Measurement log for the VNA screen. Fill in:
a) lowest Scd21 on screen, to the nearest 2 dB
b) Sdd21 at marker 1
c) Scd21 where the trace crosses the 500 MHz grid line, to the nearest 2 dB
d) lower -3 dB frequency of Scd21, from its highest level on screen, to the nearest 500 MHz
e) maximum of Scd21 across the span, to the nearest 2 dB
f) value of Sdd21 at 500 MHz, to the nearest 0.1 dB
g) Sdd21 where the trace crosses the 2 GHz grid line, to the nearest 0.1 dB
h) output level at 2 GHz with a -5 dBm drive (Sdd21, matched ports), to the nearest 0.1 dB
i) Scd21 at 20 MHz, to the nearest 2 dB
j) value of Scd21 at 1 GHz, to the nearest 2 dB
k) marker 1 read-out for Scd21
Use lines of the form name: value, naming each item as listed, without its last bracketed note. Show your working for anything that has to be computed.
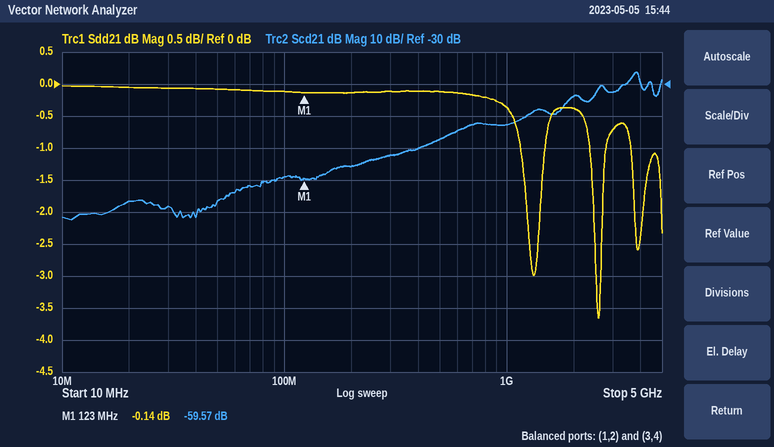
lowest Scd21 on screen, to the nearest 2 dB: -72 dB
Sdd21 at marker 1: -0.14 dB
Scd21 where the trace crosses the 500 MHz grid line, to the nearest 2 dB: -48 dB
lower -3 dB frequency of Scd21, from its highest level on screen, to the nearest 500 MHz: 3.5 GHz
maximum of Scd21 across the span, to the nearest 2 dB: -26 dB
value of Sdd21 at 500 MHz, to the nearest 0.1 dB: -0.1 dB
Sdd21 where the trace crosses the 2 GHz grid line, to the nearest 0.1 dB: -0.4 dB
output level at 2 GHz with a -5 dBm drive (Sdd21, matched ports), to the nearest 0.1 dB: -5 dBm + (-0.4 dB) = -5.4 dBm
Scd21 at 20 MHz, to the nearest 2 dB: -66 dB
value of Scd21 at 1 GHz, to the nearest 2 dB: -42 dB
marker 1 read-out for Scd21: -59.57 dB
